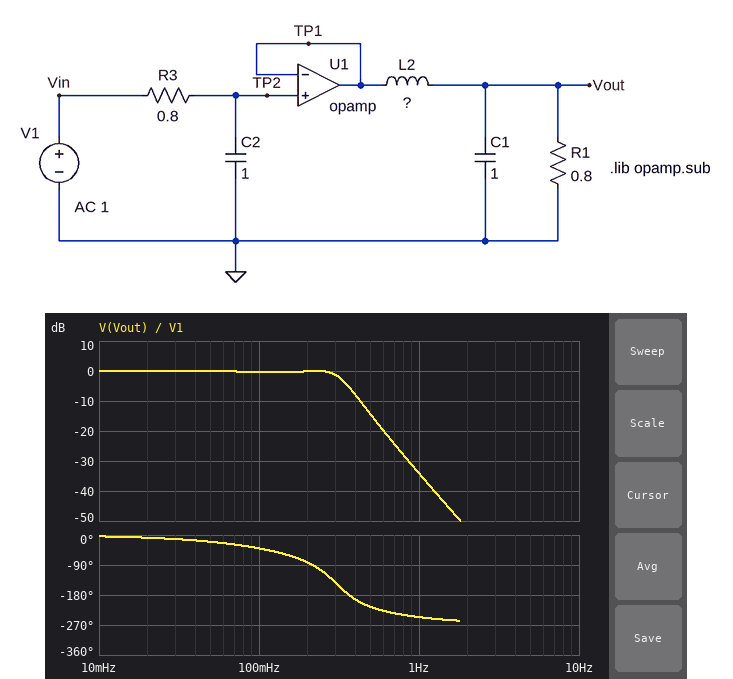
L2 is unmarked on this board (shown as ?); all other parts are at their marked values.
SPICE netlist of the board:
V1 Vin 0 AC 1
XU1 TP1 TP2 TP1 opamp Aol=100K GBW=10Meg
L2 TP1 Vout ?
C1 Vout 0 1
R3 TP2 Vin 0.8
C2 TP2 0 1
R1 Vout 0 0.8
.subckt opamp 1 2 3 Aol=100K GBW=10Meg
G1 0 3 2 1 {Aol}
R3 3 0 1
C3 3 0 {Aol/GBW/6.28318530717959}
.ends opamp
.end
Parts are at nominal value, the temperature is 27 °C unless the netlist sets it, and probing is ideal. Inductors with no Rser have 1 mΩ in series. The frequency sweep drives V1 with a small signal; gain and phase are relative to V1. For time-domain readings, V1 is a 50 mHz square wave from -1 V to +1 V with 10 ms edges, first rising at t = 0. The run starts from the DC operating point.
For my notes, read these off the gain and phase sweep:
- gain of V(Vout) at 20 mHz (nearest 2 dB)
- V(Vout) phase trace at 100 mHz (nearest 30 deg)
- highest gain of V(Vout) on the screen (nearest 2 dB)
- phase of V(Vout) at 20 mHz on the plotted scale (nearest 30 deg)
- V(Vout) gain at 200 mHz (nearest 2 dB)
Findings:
0 dB
-30 deg
0 dB
0 deg
0 dB
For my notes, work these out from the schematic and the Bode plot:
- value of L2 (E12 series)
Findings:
270 mH
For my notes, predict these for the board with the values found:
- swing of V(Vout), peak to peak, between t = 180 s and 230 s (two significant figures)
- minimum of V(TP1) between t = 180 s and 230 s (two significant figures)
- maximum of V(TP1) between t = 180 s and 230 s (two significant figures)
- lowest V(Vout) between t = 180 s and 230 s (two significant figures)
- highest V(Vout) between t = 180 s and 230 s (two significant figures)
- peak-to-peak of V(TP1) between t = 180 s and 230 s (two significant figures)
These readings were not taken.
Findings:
2.4 V
-1.0 V
1.0 V
-1.2 V
1.2 V
2.0 V
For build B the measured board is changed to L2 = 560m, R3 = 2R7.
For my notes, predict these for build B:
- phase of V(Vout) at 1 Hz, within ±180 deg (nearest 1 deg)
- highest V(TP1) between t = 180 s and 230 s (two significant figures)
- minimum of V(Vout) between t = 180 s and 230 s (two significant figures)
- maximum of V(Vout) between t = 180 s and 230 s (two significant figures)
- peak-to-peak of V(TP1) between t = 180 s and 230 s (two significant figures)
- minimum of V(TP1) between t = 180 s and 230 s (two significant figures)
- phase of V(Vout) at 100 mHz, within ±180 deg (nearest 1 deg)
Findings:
105 deg
950 mV
-940 mV
940 mV
1.9 V
-950 mV
-89 deg
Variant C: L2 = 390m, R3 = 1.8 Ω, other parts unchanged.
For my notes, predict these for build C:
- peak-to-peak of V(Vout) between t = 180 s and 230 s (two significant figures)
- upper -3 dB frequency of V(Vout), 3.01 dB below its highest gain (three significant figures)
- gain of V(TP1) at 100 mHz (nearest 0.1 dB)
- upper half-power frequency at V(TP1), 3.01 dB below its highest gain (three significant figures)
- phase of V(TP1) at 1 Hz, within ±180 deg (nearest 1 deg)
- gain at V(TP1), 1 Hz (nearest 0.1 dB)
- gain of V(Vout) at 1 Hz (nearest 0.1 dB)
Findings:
2.0 V
112 mHz
-3.6 dB
88.4 mHz
-85 deg
-21.1 dB
-44.5 dB
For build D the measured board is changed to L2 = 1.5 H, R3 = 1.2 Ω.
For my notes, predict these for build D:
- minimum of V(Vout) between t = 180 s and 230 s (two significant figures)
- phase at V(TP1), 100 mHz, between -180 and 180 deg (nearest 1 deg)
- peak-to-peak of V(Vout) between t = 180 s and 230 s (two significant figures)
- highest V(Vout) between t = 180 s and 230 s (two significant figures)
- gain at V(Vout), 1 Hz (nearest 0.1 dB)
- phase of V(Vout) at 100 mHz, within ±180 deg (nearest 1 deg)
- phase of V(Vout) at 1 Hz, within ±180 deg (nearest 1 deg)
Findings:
-1.0 V
-37 deg
2.0 V
1.0 V
-53.1 dB
-108 deg
109 deg
